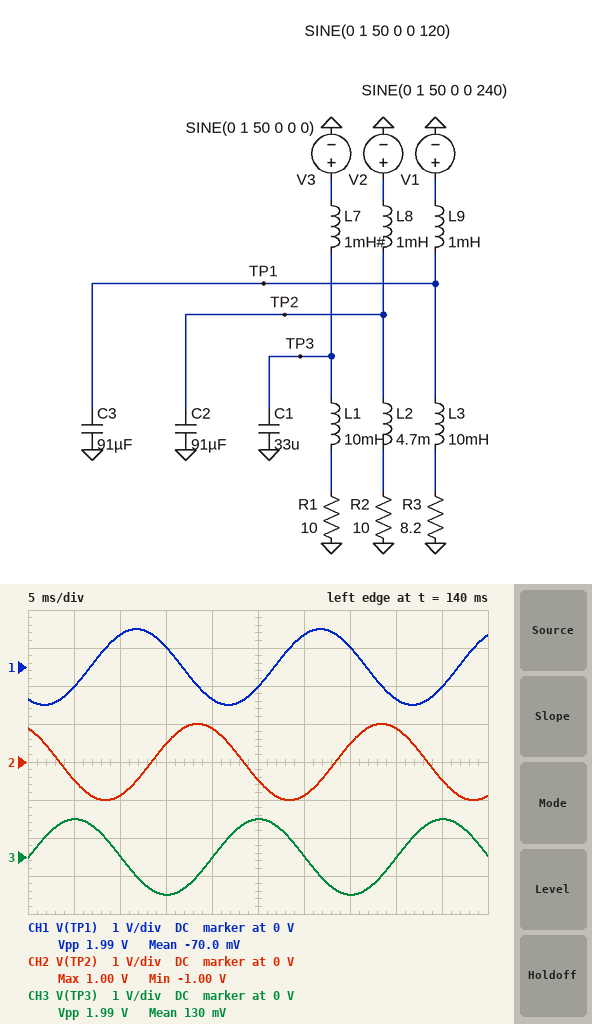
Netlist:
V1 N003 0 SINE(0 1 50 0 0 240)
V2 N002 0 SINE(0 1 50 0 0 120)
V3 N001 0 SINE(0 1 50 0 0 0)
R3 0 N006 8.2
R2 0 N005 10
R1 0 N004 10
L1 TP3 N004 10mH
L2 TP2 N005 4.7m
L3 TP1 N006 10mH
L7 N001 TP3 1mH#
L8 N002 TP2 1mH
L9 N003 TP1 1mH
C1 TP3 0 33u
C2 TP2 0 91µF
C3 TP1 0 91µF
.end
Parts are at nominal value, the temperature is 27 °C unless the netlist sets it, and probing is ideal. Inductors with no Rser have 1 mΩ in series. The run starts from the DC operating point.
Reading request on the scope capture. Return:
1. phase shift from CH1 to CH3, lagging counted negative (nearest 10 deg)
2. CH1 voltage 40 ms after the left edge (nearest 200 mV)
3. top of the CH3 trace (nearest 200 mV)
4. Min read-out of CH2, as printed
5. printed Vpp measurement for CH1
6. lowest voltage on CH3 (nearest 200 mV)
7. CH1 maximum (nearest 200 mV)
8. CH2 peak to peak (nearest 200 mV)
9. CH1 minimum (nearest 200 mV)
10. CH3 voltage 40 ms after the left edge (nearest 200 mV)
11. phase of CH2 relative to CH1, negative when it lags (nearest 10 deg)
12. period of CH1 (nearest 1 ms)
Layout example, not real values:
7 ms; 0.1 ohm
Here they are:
120 deg; -800 mV; 1.0 V; -1.00 V; 1.99 V; -1.0 V; 1.0 V; 2.0 V; -1.0 V; 0 V; -120 deg; 20 ms
